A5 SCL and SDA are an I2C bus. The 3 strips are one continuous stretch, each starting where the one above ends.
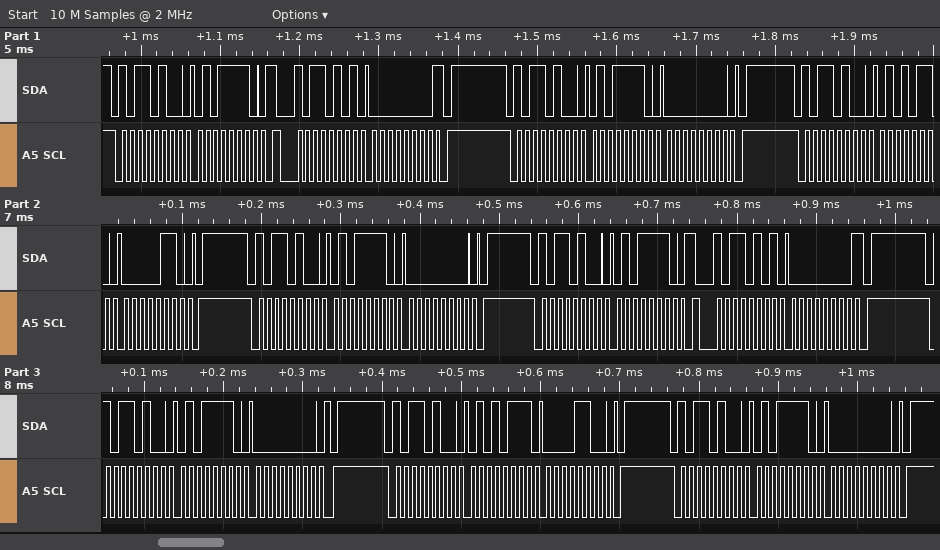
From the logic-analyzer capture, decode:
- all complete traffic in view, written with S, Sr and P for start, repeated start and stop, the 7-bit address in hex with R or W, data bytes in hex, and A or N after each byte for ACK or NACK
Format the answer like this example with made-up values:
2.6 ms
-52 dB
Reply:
S 5AW A 5E A Sr 5AR A 00 N P S 5AW A 5E A 00 A P S 5AW A 56 A 06 A P S 5AW A 5E A 00 A P S 5AW A 5E A Sr 5AR A 00 N P S 5AW A 5E A 00 A P S 5AW A 57 A 0C A P S 5AW A 5E A 00 A P
